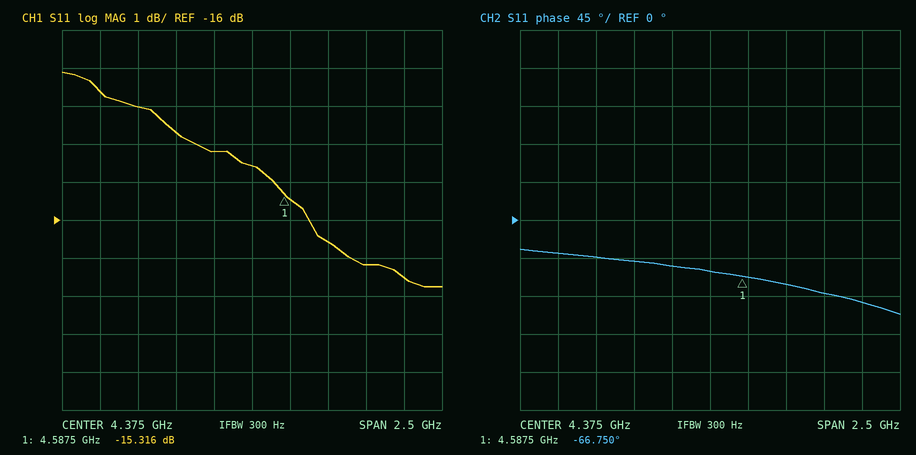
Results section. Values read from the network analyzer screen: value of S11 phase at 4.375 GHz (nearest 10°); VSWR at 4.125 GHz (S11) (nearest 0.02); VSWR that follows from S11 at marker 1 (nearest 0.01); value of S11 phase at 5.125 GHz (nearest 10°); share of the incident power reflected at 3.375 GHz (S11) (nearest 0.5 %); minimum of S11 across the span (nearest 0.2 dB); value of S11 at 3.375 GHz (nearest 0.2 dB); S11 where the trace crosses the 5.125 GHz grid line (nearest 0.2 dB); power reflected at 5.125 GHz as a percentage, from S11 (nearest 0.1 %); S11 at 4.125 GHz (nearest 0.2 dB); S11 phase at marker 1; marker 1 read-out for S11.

-60°
1.48
1.41
-90°
5.5 %
-17.8 dB
-12.6 dB
-17.2 dB
1.9 %
-14.2 dB
-66.750°
-15.316 dB
